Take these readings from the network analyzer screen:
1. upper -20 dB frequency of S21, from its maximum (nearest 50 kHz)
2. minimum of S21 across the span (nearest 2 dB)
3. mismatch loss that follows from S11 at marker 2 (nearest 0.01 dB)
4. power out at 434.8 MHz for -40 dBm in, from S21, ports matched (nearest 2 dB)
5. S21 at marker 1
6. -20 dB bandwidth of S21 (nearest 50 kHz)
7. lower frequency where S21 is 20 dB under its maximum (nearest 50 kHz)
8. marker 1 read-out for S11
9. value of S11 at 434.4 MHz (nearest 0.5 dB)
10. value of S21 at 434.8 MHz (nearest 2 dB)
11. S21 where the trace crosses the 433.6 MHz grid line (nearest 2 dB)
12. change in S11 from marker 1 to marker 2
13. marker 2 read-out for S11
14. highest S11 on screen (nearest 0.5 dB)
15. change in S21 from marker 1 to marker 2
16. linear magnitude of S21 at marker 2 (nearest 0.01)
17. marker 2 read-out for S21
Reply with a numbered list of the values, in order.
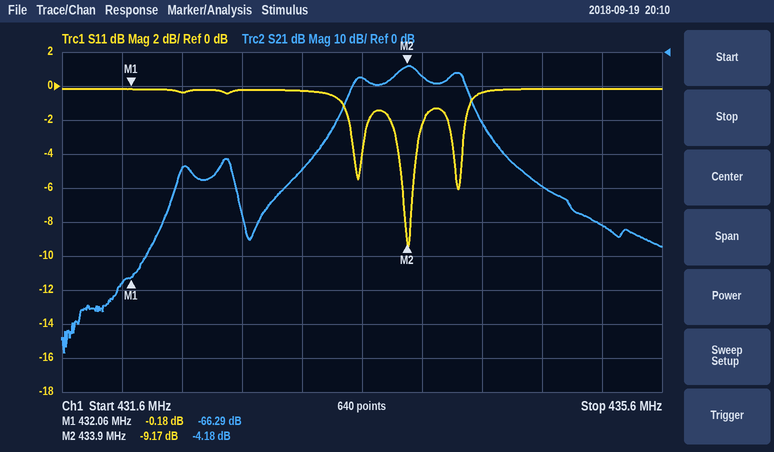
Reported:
1. 434.45 MHz
2. -88 dB
3. 0.56 dB
4. -80 dBm
5. -66.29 dB
6. 1.05 MHz
7. 433.40 MHz
8. -0.18 dB
9. -0.5 dB
10. -40 dB
11. -8 dB
12. -8.99 dB
13. -9.17 dB
14. 0.0 dB
15. 62.11 dB
16. 0.62
17. -4.18 dB
